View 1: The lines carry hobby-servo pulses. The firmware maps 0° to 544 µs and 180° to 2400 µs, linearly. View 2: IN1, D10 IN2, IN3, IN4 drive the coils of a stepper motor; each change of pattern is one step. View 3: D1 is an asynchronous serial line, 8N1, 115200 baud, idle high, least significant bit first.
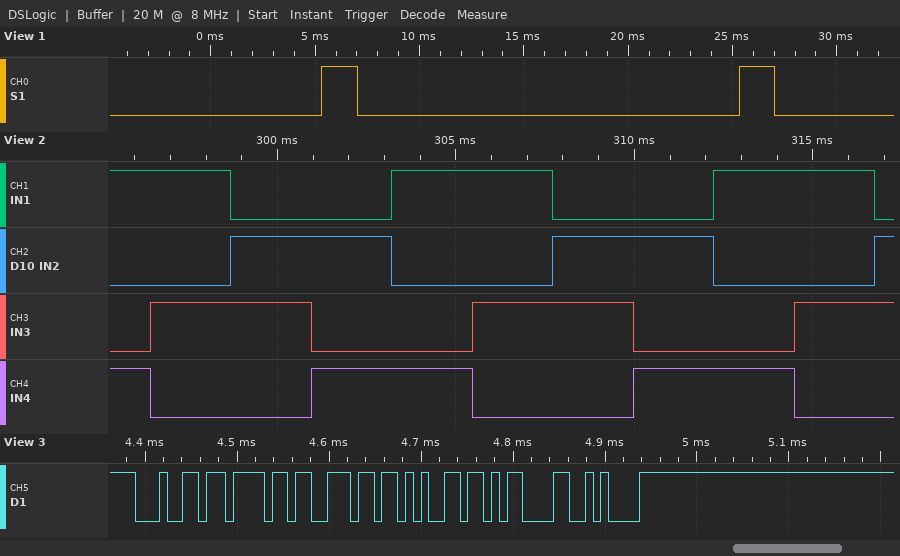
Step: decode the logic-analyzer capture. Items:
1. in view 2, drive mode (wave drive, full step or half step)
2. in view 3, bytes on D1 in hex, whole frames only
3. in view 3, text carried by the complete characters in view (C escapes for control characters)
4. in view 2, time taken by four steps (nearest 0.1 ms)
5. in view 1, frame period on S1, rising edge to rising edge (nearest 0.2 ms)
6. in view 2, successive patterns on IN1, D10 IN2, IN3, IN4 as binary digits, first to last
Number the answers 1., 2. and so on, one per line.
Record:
1. full step
2. 64 6F 6E 65 0D 0A
3. "done\r\n"
4. 9.0 ms
5. 20.0 ms
6. 1001 1010 0110 0101 1001 1010 0110 0101 1001 1010 0110
